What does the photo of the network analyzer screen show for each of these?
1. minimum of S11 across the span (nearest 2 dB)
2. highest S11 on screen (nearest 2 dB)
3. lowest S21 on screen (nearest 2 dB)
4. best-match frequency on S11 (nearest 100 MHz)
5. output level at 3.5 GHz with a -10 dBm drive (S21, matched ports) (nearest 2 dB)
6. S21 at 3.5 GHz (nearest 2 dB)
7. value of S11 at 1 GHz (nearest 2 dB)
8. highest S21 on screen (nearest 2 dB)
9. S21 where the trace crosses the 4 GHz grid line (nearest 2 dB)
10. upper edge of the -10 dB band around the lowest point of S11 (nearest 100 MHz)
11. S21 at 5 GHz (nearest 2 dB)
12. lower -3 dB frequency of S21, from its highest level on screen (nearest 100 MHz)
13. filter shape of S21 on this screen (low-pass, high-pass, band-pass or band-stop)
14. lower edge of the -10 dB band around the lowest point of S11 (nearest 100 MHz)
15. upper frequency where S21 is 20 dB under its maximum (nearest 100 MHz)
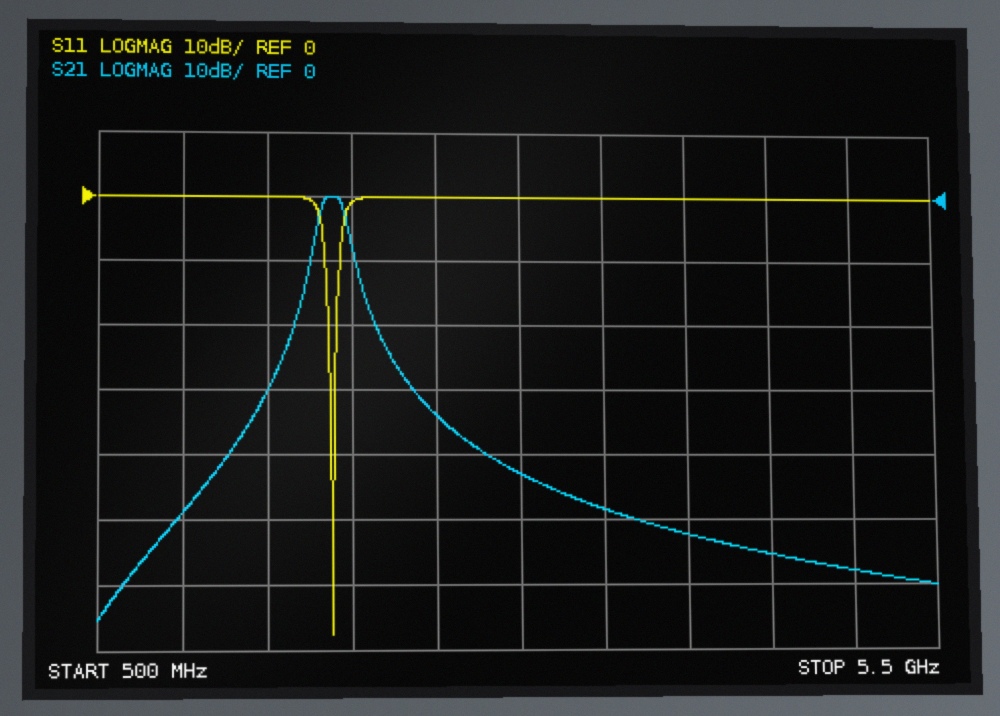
-68 dB
0 dB
-66 dB
1.9 GHz
-58 dBm
-48 dB
0 dB
0 dB
-52 dB
1.9 GHz
-58 dB
1.8 GHz
band-pass
1.8 GHz
2.1 GHz
